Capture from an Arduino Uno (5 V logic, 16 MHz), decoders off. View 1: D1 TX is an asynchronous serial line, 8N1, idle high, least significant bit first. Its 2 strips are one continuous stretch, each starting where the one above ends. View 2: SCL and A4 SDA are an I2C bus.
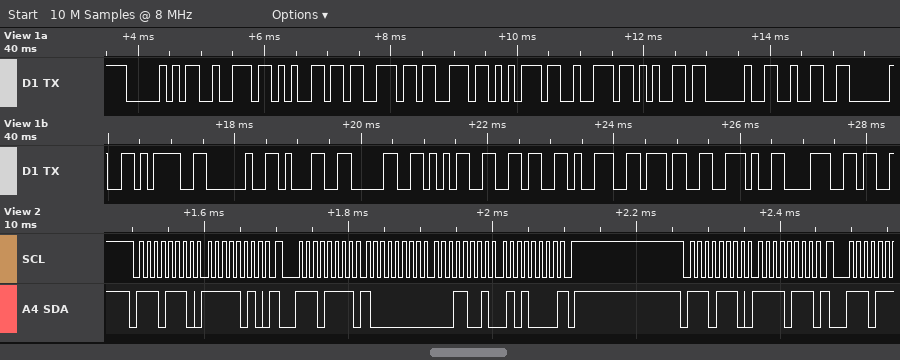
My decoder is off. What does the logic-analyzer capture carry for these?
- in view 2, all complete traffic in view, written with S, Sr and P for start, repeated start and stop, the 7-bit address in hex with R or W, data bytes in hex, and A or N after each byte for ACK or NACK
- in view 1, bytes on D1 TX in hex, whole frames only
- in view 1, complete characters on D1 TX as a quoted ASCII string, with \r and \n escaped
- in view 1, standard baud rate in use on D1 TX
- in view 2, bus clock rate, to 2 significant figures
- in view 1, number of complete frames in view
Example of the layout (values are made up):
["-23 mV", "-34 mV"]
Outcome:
["S 77W A FA A Sr 77R A 80 A 19 A 50 N P S 77W A F7 A", "0x50 0x72 0x65 0x73 0x73 0x75 0x72 0x65 0x20 0x32 0x20 0x3D 0x20 0x31 0x30 0x35 0x36 0x39 0x37 0x2E 0x38", "\"Pressure 2 = 105697.8\"", "9600 baud", "100 kHz", "21"]
